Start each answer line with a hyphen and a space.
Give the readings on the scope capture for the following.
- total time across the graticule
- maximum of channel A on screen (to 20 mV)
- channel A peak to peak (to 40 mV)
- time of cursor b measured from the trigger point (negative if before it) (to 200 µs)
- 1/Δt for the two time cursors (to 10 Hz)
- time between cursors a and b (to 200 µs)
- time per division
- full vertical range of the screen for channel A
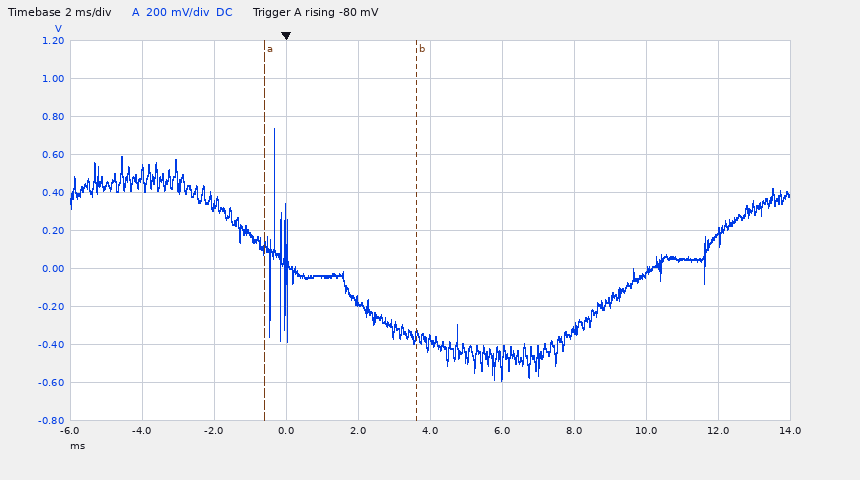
- 20 ms
- 740 mV
- 1.32 V
- +3.6 ms
- 240 Hz
- 4.2 ms
- 2 ms
- 2 V
